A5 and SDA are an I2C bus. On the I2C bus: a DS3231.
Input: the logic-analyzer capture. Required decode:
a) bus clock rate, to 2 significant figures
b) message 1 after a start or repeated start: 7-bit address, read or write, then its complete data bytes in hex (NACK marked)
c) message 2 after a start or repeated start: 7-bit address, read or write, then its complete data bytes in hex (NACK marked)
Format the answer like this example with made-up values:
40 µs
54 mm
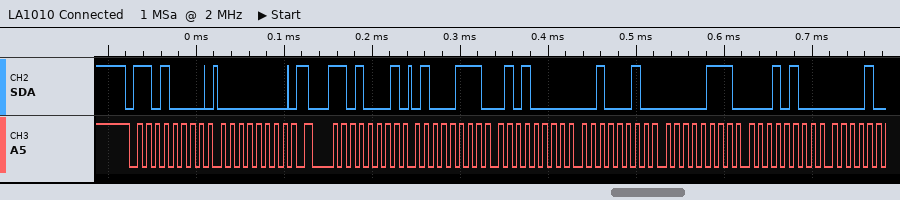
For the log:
100 kHz
0x68 write: 00
0x68 read: 47 50 22 07 14
